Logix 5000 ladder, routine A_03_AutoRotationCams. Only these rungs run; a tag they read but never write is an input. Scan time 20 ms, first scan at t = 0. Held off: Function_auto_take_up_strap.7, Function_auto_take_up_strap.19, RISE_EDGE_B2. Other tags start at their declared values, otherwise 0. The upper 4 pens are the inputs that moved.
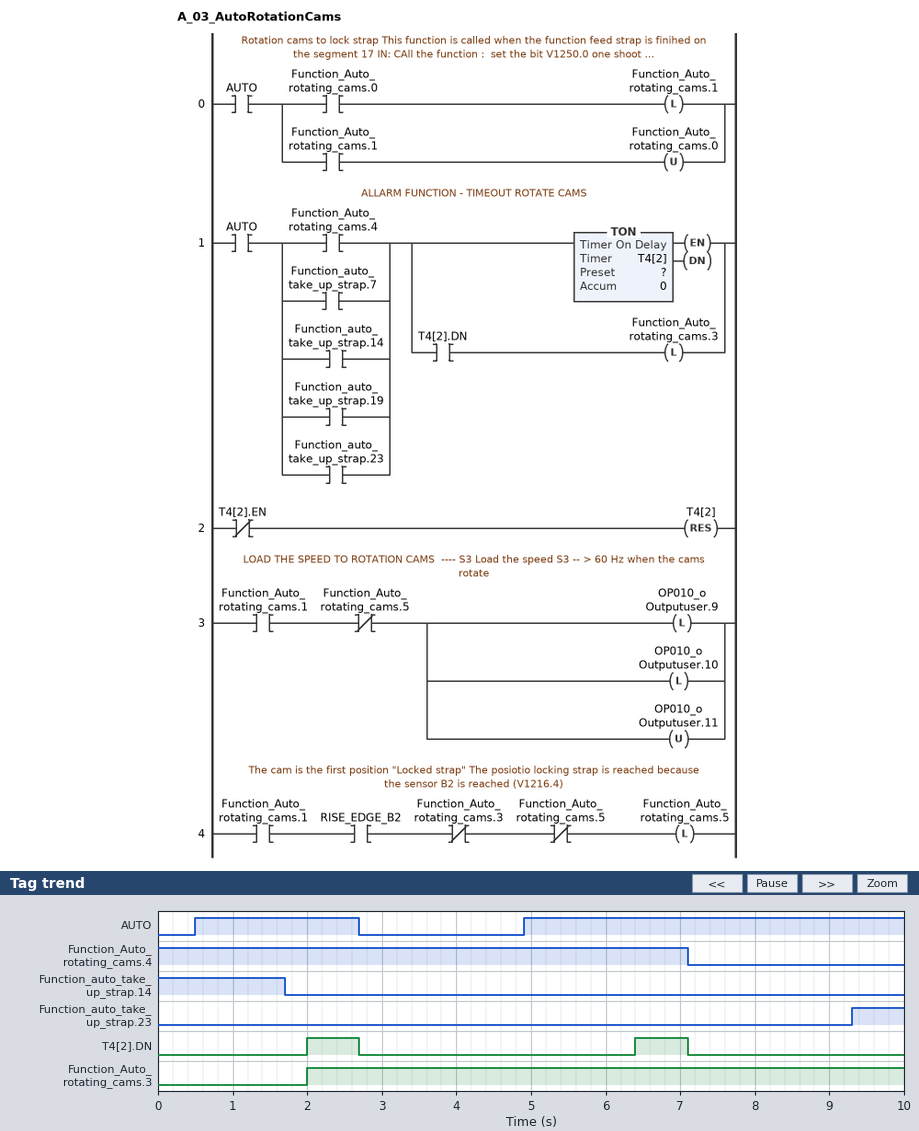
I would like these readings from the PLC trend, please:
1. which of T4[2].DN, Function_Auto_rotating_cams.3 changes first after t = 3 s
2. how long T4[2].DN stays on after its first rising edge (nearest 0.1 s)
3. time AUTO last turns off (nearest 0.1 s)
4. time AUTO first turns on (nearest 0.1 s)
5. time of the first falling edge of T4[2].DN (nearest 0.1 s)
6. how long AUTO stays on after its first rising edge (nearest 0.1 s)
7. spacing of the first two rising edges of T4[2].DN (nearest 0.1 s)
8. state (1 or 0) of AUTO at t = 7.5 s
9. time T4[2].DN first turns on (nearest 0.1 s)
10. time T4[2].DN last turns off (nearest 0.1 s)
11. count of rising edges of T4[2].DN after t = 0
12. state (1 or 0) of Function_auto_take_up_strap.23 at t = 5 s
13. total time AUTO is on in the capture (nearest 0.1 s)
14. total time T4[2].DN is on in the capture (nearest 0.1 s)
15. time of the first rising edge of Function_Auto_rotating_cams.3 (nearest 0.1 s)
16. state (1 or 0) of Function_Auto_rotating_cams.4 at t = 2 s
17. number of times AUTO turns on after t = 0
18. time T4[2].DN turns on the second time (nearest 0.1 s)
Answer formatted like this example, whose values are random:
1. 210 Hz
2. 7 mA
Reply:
1. T4[2].DN
2. 0.7 s
3. 2.7 s
4. 0.5 s
5. 2.7 s
6. 2.2 s
7. 4.4 s
8. 1
9. 2.0 s
10. 7.1 s
11. 2
12. 0
13. 7.3 s
14. 1.4 s
15. 2.0 s
16. 1
17. 2
18. 6.4 s
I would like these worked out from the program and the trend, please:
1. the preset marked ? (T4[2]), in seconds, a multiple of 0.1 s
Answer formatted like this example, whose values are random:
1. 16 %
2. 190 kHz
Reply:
1. 1.5 s
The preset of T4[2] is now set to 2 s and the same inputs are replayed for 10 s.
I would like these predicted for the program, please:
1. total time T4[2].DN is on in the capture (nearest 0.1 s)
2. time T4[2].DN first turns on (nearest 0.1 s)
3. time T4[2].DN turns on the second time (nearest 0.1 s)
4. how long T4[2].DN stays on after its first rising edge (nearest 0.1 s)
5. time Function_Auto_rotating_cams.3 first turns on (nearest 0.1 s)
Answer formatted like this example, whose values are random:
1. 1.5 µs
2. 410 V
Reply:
1. 0.4 s
2. 2.5 s
3. 6.9 s
4. 0.2 s
5. 2.5 s
